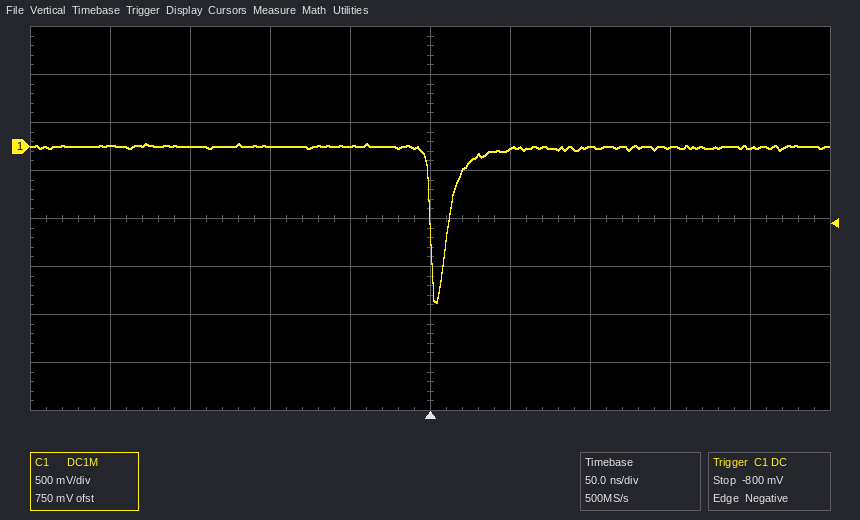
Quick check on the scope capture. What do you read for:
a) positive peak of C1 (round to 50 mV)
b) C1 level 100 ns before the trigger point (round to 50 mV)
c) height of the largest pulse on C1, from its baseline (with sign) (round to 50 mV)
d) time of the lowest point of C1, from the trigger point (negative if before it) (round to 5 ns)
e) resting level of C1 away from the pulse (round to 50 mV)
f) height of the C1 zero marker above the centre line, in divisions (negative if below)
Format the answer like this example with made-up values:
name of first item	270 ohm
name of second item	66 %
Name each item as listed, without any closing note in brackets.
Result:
positive peak of C1	50 mV
C1 level 100 ns before the trigger point	0 mV
height of the largest pulse on C1, from its baseline (with sign)	-1.60 V
time of the lowest point of C1, from the trigger point (negative if before it)	+5 ns
resting level of C1 away from the pulse	0 mV
height of the C1 zero marker above the centre line, in divisions	+1.5 div
